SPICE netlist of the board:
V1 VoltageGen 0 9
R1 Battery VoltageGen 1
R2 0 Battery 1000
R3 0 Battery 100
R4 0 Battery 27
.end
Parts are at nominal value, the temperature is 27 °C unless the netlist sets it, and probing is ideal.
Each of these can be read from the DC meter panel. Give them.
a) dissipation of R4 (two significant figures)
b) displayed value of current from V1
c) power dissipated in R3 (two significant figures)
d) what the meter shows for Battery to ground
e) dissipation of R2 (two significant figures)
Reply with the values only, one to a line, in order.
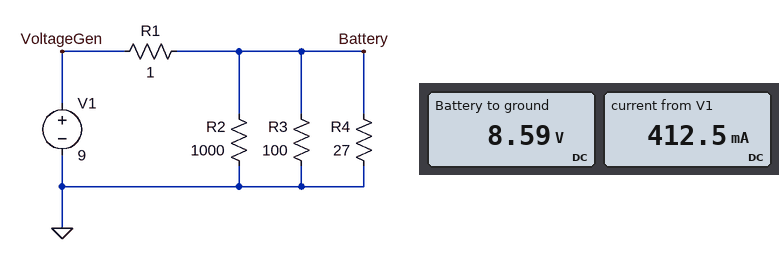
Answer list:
2.7 W
412.5 mA
740 mW
8.59 V
74 mW
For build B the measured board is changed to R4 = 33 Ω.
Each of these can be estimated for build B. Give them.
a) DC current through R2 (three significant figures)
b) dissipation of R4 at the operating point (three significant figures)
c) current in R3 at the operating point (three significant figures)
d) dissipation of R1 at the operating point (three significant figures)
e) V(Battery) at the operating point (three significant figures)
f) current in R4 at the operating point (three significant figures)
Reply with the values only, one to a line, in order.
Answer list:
8.64 mA
2.26 W
86.4 mA
127 mW
8.64 V
262 mA
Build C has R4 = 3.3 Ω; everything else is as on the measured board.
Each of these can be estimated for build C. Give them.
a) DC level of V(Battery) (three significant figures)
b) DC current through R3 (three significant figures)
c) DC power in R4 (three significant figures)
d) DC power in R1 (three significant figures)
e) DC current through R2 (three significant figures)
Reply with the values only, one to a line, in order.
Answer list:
6.85 V
68.5 mA
14.2 W
4.63 W
6.85 mA
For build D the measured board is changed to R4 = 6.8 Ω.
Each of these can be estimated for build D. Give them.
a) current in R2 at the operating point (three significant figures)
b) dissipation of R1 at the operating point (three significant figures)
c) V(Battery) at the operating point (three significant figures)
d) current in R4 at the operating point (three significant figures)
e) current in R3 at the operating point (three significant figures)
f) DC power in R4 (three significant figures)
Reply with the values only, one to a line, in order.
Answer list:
7.77 mA
1.51 W
7.77 V
1.14 A
77.7 mA
8.88 W
